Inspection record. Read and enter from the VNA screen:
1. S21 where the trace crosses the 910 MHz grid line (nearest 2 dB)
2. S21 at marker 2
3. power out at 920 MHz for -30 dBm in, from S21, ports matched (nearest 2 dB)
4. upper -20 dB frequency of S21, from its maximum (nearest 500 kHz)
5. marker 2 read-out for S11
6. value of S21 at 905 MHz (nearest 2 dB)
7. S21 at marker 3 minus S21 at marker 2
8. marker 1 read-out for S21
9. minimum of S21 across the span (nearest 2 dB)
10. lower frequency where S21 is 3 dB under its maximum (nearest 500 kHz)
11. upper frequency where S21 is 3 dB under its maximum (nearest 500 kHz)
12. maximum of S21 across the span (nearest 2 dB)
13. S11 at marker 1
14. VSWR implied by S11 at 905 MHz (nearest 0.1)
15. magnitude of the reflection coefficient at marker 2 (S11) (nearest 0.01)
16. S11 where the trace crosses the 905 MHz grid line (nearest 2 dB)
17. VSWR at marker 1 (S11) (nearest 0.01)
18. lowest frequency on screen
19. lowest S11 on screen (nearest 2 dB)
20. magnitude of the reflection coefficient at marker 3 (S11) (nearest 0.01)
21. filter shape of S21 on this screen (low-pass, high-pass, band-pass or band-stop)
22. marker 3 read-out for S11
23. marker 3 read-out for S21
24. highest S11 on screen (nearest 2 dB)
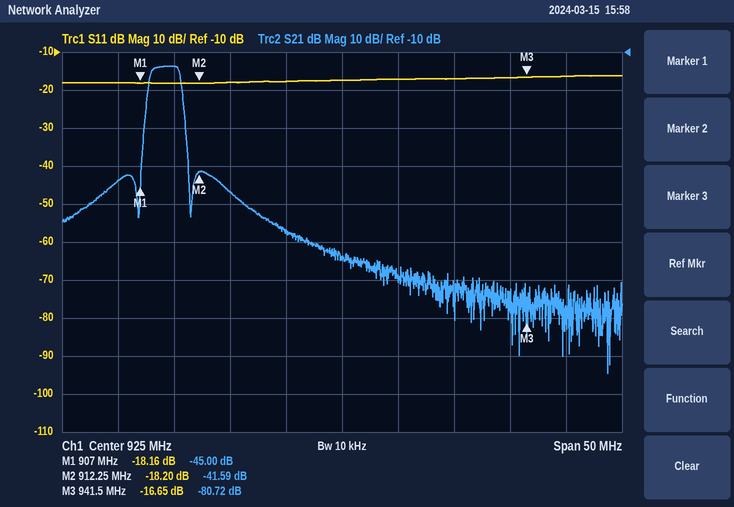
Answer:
-14 dB
-41.59 dB
-88 dBm
911.0 MHz
-18.20 dB
-44 dB
-39.13 dB
-45.00 dB
-94 dB
908.0 MHz
910.5 MHz
-14 dB
-18.16 dB
1.3
0.12
-18 dB
1.28
900 MHz
-18 dB
0.15
band-pass
-16.65 dB
-80.72 dB
-16 dB
